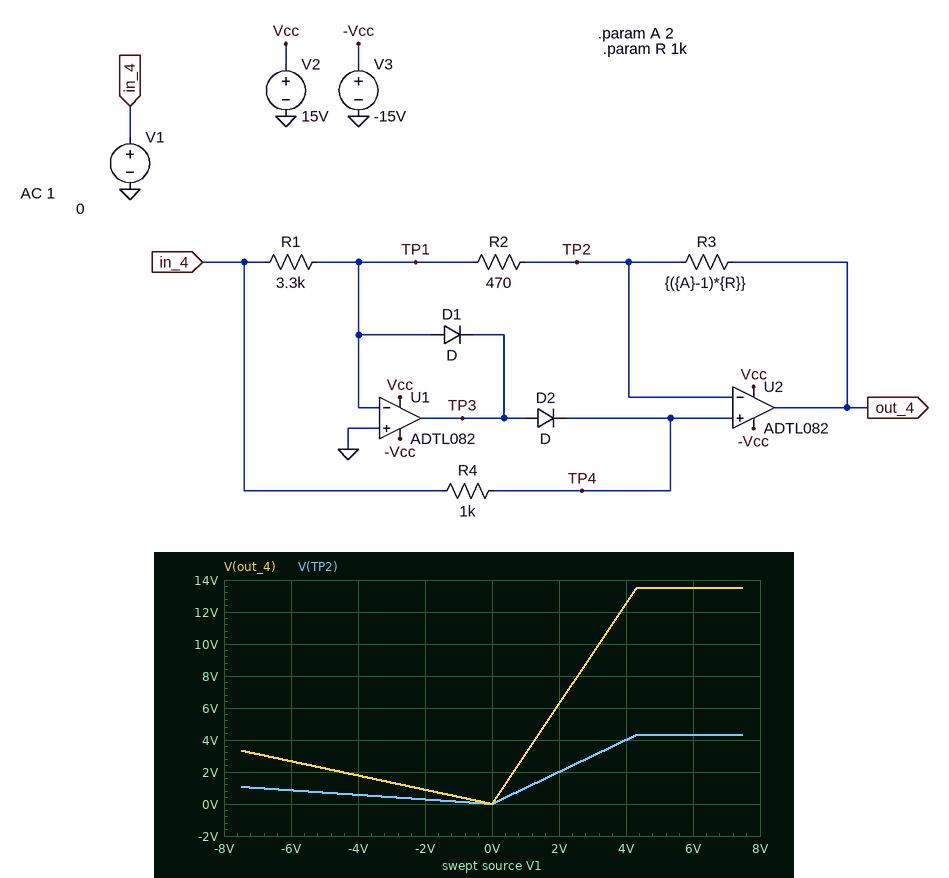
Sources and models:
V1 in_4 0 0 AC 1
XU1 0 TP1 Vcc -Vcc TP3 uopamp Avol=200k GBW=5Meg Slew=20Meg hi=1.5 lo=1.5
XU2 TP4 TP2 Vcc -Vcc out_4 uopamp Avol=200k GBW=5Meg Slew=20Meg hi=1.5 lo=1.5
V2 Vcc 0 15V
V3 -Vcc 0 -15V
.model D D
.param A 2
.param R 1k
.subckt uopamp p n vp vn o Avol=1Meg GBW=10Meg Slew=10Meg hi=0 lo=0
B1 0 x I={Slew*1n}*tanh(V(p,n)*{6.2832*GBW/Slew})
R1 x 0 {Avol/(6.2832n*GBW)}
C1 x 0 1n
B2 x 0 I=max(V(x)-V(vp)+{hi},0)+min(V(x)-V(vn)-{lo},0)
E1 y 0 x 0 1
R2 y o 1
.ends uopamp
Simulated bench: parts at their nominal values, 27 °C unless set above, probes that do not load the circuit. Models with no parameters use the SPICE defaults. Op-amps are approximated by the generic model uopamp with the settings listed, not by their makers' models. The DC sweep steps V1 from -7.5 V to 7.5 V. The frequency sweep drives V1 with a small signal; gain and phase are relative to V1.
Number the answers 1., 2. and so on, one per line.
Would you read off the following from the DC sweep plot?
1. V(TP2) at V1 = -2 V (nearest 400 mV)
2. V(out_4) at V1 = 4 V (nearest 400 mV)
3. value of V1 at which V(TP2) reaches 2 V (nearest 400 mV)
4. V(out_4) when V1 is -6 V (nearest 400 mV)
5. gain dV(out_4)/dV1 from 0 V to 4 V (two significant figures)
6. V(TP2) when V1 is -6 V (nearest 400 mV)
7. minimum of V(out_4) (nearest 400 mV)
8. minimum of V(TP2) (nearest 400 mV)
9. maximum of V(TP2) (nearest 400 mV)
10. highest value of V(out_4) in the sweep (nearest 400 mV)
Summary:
1. 400 mV
2. 12.4 V
3. 2.0 V
4. 2.8 V
5. 3.1 V/V
6. 800 mV
7. 0 V
8. 0 V
9. 4.4 V
10. 13.6 V
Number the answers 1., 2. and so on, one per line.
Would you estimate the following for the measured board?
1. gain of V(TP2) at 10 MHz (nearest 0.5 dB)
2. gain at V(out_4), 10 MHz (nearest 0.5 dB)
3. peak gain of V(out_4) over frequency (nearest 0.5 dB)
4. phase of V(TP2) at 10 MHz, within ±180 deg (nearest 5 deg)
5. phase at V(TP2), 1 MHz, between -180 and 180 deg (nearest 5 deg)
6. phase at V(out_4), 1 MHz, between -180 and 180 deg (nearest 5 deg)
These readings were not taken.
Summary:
1. -7.5 dB
2. -8.5 dB
3. 0 dB
4. -40 deg
5. -10 deg
6. -15 deg
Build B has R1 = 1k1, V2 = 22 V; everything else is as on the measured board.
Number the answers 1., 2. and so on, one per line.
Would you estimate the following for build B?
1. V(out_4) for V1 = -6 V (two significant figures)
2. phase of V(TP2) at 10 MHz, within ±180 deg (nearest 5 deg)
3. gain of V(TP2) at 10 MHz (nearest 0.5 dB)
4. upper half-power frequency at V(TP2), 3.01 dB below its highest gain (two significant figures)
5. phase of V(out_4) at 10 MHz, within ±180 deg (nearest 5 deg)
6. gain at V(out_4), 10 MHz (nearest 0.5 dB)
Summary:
1. 8.0 V
2. -20 deg
3. -6.5 dB
4. 3.7 MHz
5. -75 deg
6. -10.5 dB
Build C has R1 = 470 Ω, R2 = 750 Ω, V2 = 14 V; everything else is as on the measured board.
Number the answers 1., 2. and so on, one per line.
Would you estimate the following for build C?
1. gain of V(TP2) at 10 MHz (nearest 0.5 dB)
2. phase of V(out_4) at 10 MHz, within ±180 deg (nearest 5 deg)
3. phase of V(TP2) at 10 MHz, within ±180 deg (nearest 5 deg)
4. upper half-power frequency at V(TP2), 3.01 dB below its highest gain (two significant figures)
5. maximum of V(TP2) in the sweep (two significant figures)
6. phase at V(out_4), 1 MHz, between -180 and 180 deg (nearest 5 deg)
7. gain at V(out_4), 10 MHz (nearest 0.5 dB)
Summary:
1. -6.0 dB
2. -75 deg
3. -15 deg
4. 3.6 MHz
5. 5.4 V
6. -20 deg
7. -11.5 dB
